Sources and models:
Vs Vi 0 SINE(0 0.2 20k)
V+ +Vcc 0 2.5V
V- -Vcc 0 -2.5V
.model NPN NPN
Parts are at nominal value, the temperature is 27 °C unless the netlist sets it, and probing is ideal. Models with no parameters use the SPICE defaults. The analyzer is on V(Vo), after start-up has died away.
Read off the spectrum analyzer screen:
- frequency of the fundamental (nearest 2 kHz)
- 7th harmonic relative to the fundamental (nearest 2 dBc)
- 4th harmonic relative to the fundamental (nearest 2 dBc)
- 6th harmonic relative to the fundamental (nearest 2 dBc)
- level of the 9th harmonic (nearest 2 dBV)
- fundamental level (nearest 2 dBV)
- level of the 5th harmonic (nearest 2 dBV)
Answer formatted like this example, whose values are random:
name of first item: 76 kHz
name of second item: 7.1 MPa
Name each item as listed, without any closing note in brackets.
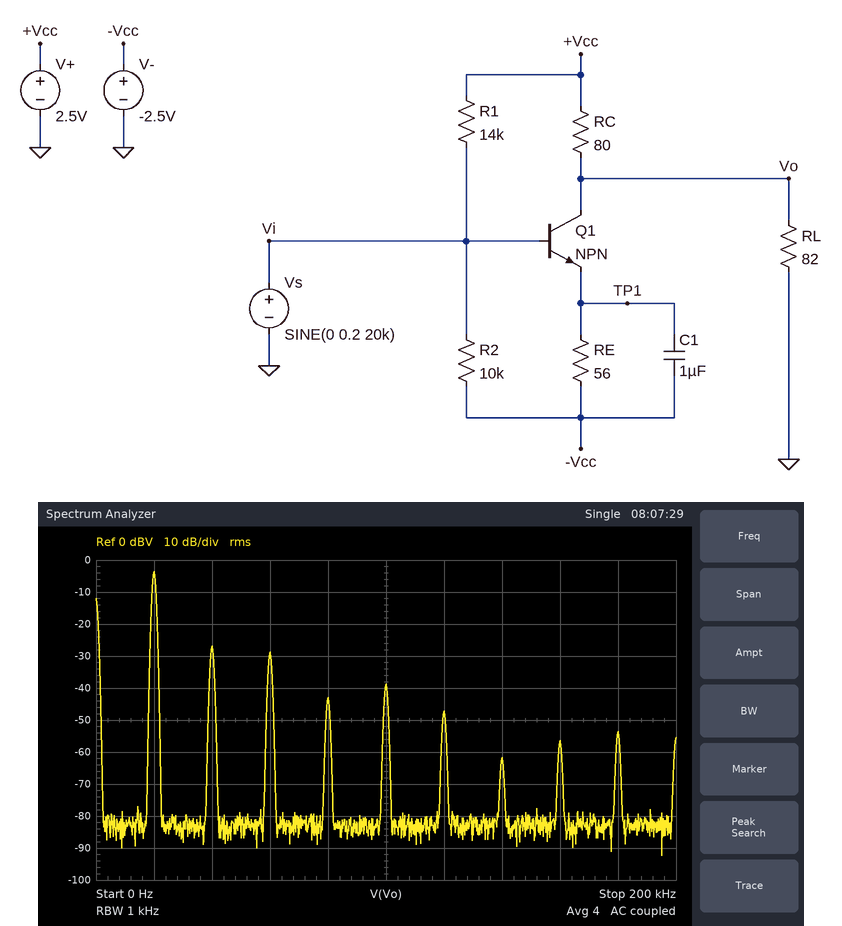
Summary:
frequency of the fundamental: 20 kHz
7th harmonic relative to the fundamental: -58 dBc
4th harmonic relative to the fundamental: -40 dBc
6th harmonic relative to the fundamental: -44 dBc
level of the 9th harmonic: -54 dBV
fundamental level: -4 dBV
level of the 5th harmonic: -38 dBV
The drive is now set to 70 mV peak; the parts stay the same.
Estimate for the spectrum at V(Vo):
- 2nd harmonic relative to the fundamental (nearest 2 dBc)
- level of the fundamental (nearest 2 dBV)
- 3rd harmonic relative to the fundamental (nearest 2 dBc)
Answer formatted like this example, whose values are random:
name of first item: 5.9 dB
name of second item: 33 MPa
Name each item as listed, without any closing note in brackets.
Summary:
2nd harmonic relative to the fundamental: -36 dBc
level of the fundamental: -12 dBV
3rd harmonic relative to the fundamental: -52 dBc
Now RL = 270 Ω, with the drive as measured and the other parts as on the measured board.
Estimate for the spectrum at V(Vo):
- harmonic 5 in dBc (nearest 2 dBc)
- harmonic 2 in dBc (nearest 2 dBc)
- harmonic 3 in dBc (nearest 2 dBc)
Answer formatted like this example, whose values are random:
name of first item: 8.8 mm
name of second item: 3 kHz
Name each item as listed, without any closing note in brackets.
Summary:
harmonic 5 in dBc: -44 dBc
harmonic 2 in dBc: -18 dBc
harmonic 3 in dBc: -20 dBc
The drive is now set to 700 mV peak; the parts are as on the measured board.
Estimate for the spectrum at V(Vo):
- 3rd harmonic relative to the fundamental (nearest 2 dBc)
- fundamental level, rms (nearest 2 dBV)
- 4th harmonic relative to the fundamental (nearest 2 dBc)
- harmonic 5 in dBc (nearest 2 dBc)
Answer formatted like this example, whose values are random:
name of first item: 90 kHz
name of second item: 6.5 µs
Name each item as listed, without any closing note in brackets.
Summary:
3rd harmonic relative to the fundamental: -12 dBc
fundamental level, rms: -2 dBV
4th harmonic relative to the fundamental: -12 dBc
harmonic 5 in dBc: -20 dBc
